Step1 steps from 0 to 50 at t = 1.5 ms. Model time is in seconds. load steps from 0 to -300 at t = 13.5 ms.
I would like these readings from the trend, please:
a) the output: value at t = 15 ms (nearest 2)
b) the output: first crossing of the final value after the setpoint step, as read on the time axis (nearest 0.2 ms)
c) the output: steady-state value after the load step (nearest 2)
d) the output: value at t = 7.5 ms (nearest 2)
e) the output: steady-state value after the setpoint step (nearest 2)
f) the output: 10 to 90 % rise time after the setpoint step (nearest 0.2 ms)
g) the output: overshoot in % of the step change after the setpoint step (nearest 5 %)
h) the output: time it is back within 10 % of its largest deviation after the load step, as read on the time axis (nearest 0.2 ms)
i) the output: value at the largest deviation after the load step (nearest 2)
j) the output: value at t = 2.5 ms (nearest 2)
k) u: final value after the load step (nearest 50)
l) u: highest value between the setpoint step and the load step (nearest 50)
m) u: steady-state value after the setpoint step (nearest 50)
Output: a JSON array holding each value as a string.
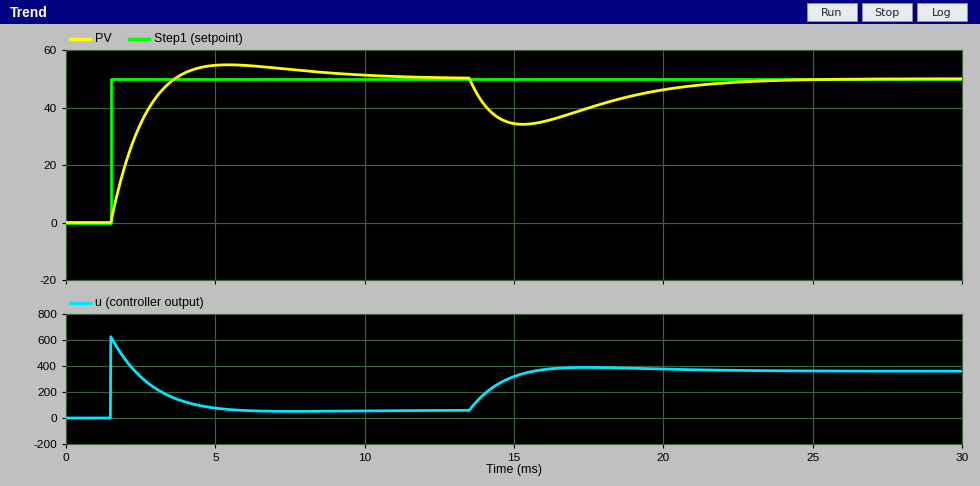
["34", "3.6 ms", "50", "54", "50", "1.6 ms", "10 %", "21.8 ms", "34", "34", "350", "600", "50"]
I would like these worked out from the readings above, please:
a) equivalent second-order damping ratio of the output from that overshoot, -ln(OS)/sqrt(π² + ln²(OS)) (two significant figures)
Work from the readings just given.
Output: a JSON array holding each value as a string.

["0.59"]
